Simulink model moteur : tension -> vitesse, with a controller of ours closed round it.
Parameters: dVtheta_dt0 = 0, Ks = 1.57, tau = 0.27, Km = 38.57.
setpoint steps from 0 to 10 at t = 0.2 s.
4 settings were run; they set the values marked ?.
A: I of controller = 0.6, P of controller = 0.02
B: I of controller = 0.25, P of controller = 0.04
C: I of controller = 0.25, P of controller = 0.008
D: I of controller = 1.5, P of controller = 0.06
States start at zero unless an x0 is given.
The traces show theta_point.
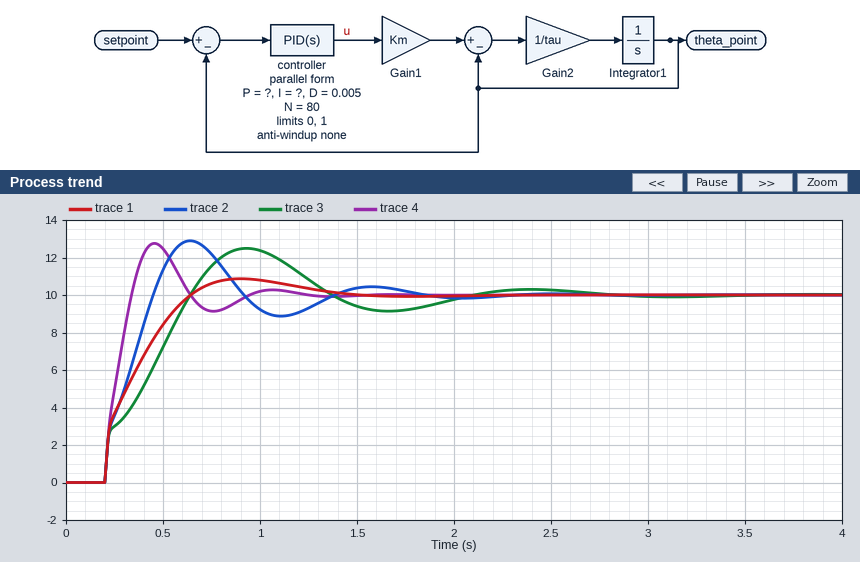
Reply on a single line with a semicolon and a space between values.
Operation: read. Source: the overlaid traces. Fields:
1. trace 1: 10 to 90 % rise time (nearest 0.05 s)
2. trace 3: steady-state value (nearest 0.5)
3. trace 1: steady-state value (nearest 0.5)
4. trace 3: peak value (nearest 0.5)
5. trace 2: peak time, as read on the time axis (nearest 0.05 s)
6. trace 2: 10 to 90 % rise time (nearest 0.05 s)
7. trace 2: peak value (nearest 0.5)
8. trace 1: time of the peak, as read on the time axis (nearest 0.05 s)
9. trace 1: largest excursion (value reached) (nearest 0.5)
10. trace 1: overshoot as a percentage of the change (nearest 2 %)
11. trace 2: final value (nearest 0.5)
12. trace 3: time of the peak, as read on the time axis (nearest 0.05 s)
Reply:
0.35 s; 10.0; 10.0; 12.5; 0.65 s; 0.20 s; 13.0; 0.90 s; 11.0; 8 %; 10.0; 0.95 s
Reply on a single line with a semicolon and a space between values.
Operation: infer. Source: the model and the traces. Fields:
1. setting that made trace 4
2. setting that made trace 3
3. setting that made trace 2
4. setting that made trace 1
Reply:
D; C; A; B
